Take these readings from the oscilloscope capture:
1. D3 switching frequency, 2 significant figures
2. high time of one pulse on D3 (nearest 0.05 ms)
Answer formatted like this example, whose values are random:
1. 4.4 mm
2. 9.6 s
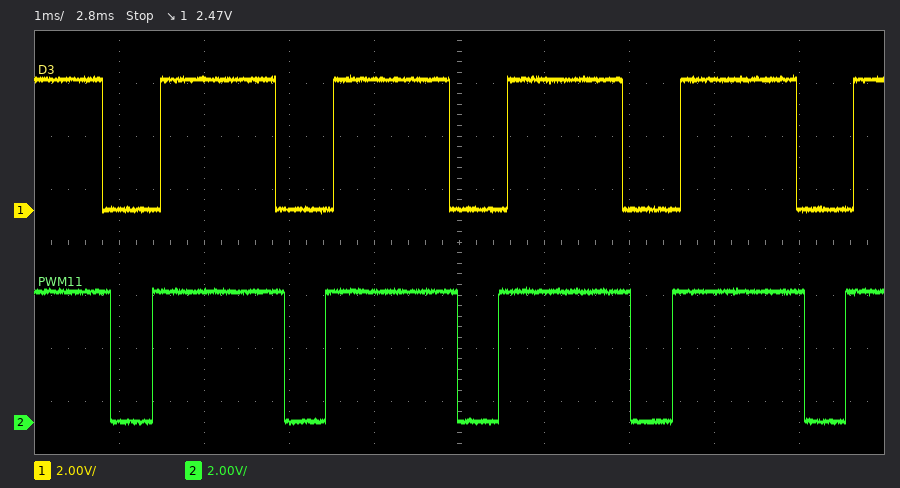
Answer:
1. 490 Hz
2. 1.35 ms
